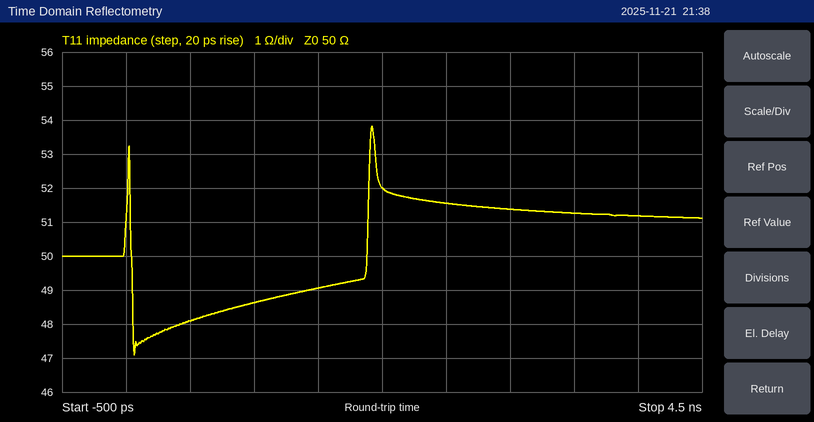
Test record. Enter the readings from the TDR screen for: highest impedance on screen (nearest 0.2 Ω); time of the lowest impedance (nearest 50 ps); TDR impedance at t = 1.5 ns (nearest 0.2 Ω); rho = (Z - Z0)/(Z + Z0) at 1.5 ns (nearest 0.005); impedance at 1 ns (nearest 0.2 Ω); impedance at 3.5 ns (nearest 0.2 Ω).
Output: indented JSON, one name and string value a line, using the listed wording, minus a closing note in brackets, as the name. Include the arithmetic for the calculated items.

{
  "highest impedance on screen": "53.8 Ω",
  "time of the lowest impedance": "50 ps",
  "TDR impedance at t = 1.5 ns": "49.0 Ω",
  "rho = (Z - Z0)/(Z + Z0) at 1.5 ns": "(49 − 50)/(49 + 50) ≈ -0.010",
  "impedance at 1 ns": "48.6 Ω",
  "impedance at 3.5 ns": "51.2 Ω"
}
